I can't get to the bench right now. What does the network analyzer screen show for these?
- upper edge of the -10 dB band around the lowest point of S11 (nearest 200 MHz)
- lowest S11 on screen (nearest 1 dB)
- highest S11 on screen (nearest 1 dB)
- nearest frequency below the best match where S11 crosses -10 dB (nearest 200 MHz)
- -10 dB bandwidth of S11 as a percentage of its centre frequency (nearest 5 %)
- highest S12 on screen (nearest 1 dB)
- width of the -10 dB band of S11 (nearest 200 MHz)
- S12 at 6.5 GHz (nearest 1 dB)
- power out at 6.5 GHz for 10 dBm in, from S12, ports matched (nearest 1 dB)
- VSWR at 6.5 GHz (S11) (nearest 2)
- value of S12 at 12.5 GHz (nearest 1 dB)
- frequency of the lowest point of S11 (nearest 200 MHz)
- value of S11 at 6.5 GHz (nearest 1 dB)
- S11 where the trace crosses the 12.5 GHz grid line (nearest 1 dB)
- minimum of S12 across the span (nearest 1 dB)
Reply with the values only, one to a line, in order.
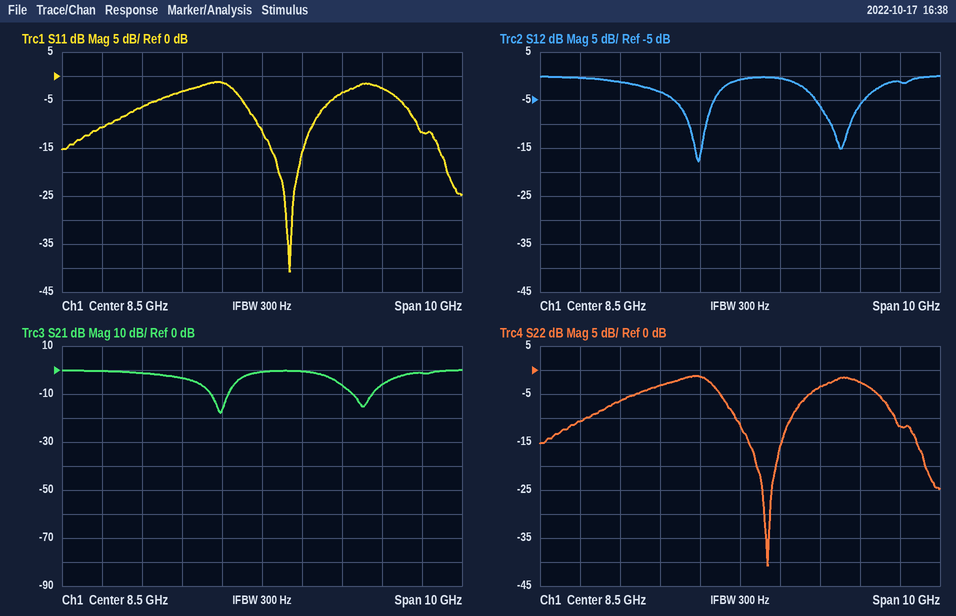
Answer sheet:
9.8 GHz
-41 dB
-1 dB
8.4 GHz
15 %
0 dB
1.4 GHz
-3 dB
7 dBm
6
-1 dB
9.2 GHz
-3 dB
-12 dB
-18 dB
